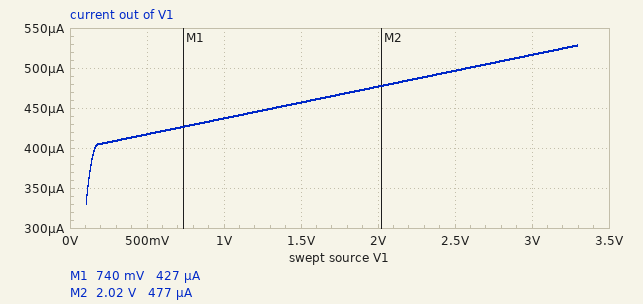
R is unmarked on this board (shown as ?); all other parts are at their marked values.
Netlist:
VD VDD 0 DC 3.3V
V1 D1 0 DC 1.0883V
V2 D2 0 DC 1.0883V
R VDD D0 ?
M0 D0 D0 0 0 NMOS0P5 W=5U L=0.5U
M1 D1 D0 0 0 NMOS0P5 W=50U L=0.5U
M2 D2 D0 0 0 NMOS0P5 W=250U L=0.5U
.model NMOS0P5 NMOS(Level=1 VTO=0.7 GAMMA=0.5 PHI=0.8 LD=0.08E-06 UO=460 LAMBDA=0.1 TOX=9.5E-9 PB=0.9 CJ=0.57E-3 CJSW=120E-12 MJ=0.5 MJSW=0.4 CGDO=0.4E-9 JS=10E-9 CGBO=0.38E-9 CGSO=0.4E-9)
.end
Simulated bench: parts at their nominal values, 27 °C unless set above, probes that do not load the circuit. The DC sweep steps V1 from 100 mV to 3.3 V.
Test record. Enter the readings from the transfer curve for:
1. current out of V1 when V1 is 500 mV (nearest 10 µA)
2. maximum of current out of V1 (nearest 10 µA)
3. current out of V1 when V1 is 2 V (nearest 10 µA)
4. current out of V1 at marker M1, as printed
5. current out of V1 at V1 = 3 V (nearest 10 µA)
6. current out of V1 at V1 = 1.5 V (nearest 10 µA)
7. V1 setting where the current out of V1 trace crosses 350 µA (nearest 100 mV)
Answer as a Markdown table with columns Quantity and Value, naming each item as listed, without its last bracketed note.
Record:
| Quantity | Value |
|---|---|
| current out of V1 when V1 is 500 mV | 420 µA |
| maximum of current out of V1 | 530 µA |
| current out of V1 when V1 is 2 V | 480 µA |
| current out of V1 at marker M1, as printed | 427 µA |
| current out of V1 at V1 = 3 V | 520 µA |
| current out of V1 at V1 = 1.5 V | 460 µA |
| V1 setting where the current out of V1 trace crosses 350 µA | 100 mV |
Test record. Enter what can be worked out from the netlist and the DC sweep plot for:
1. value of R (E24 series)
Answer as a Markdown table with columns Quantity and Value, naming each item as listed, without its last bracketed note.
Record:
| Quantity | Value |
|---|---|
| value of R | 56 kΩ |
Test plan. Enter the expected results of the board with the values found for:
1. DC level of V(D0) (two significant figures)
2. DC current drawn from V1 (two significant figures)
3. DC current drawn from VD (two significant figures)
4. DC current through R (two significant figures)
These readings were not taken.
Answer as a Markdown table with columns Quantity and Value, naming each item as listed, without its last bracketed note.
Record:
| Quantity | Value |
|---|---|
| DC level of V(D0) | 880 mV |
| DC current drawn from V1 | 440 µA |
| DC current drawn from VD | 43 µA |
| DC current through R | 43 µA |
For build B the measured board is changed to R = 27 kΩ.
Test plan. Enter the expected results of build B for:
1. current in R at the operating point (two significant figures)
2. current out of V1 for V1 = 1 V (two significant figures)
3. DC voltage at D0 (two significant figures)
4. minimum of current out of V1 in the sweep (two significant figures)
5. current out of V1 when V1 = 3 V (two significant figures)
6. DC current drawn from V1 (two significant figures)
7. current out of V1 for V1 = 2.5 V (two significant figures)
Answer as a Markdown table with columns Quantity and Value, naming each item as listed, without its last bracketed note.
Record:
| Quantity | Value |
|---|---|
| current in R at the operating point | 87 µA |
| current out of V1 for V1 = 1 V | 870 µA |
| DC voltage at D0 | 950 mV |
| minimum of current out of V1 in the sweep | 510 µA |
| current out of V1 when V1 = 3 V | 1.0 mA |
| DC current drawn from V1 | 880 µA |
| current out of V1 for V1 = 2.5 V | 990 µA |
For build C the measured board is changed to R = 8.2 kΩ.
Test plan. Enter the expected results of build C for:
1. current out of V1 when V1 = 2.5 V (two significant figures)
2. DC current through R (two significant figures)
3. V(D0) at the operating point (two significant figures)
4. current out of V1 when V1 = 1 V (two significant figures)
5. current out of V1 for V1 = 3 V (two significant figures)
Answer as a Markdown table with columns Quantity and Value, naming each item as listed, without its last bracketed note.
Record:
| Quantity | Value |
|---|---|
| current out of V1 when V1 = 2.5 V | 3.0 mA |
| DC current through R | 260 µA |
| V(D0) at the operating point | 1.1 V |
| current out of V1 when V1 = 1 V | 2.6 mA |
| current out of V1 for V1 = 3 V | 3.1 mA |
